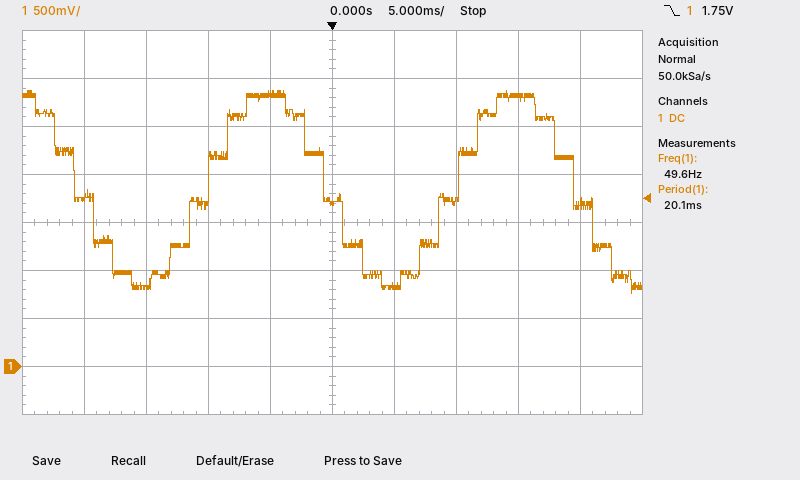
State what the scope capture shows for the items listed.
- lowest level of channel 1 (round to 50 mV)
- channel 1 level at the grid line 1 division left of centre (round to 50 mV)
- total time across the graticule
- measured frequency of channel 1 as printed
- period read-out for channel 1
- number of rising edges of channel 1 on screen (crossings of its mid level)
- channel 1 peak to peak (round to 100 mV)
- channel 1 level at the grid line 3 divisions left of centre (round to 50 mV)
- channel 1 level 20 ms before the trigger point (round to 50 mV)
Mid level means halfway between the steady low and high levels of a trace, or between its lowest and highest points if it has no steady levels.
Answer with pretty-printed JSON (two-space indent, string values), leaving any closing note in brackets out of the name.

{
  "lowest level of channel 1": "750 mV",
  "channel 1 level at the grid line 1 division left of centre": "2.85 V",
  "total time across the graticule": "50 ms",
  "measured frequency of channel 1 as printed": "49.6 Hz",
  "period read-out for channel 1": "20.1 ms",
  "number of rising edges of channel 1 on screen": "2",
  "channel 1 peak to peak": "2.10 V",
  "channel 1 level at the grid line 3 divisions left of centre": "800 mV",
  "channel 1 level 20 ms before the trigger point": "1.75 V"
}
